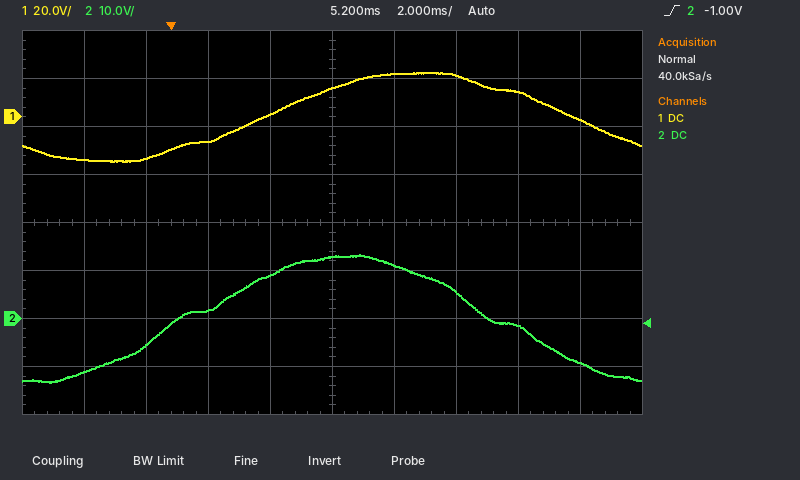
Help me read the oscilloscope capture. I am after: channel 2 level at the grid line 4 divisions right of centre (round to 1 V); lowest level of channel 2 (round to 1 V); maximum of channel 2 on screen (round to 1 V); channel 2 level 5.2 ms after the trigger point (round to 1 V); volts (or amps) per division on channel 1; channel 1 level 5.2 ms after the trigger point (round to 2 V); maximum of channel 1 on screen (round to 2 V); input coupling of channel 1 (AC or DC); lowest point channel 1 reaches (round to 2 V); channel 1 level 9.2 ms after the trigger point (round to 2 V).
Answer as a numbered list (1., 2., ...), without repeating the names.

1. -9 V
2. -13 V
3. 13 V
4. 13 V
5. 20 V
6. 12 V
7. 18 V
8. DC
9. -18 V
10. 18 V
